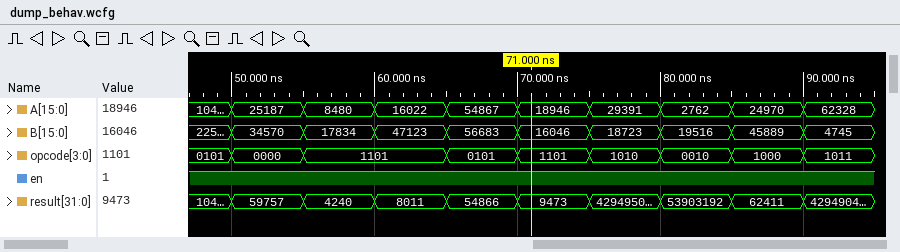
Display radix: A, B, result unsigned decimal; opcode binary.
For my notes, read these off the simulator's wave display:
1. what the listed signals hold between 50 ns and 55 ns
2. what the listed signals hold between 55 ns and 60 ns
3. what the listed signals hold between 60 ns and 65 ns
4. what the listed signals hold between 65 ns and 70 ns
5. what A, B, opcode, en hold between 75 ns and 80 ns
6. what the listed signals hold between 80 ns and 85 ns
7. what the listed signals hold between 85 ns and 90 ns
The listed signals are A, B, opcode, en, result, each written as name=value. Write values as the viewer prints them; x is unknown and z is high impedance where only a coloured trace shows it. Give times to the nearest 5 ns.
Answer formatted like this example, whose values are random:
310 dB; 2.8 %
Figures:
A=25187, B=34570, opcode=0000, en=1, result=59757; A=8480, B=17834, opcode=1101, en=1, result=4240; A=16022, B=47123, opcode=1101, en=1, result=8011; A=54867, B=56683, opcode=0101, en=1, result=54866; A=29391, B=18723, opcode=1010, en=1; A=2762, B=19516, opcode=0010, en=1, result=53903192; A=24970, B=45889, opcode=1000, en=1, result=62411
